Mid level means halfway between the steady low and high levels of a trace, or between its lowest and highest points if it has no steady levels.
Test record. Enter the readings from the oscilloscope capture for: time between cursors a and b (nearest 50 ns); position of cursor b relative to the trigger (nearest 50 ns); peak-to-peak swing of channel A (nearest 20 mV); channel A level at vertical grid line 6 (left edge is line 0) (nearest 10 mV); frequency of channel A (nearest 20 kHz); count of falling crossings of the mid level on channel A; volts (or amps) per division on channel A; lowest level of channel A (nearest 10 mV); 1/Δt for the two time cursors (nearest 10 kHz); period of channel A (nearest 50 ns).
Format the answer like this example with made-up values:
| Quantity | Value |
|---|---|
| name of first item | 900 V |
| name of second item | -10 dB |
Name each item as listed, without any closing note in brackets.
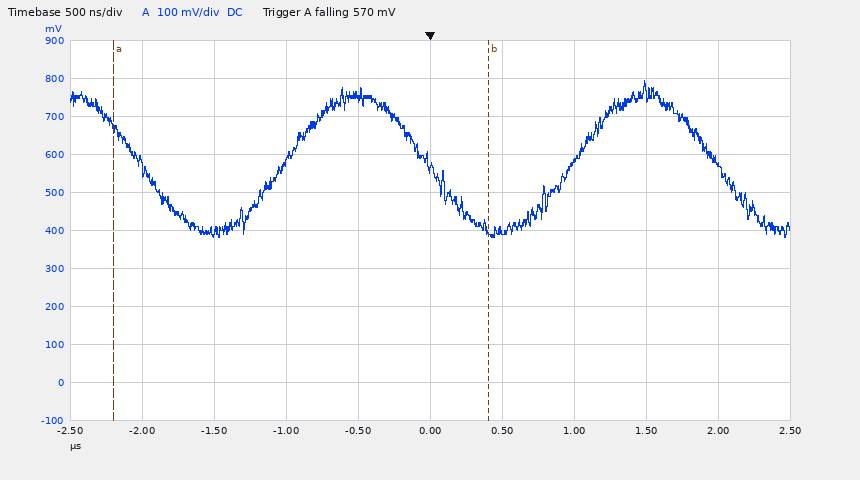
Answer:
| Quantity | Value |
|---|---|
| time between cursors a and b | 2.60 µs |
| position of cursor b relative to the trigger | +400 ns |
| peak-to-peak swing of channel A | 420 mV |
| channel A level at vertical grid line 6 (left edge is line 0) | 400 mV |
| frequency of channel A | 500 kHz |
| count of falling crossings of the mid level on channel A | 3 |
| volts (or amps) per division on channel A | 100 mV |
| lowest level of channel A | 380 mV |
| 1/Δt for the two time cursors | 380 kHz |
| period of channel A | 2.00 µs |
